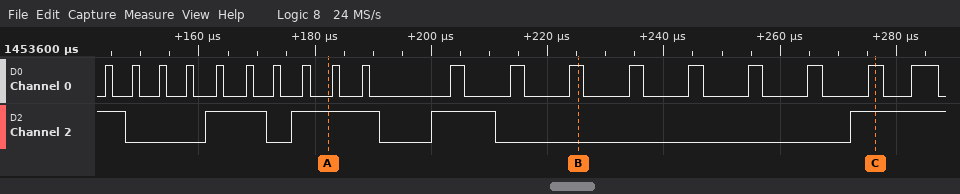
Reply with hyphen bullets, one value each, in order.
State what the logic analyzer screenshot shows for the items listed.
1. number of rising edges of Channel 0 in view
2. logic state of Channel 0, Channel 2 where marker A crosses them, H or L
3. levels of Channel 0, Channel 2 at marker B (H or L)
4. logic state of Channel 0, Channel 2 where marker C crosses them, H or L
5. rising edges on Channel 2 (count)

- 19
- Channel 0=L, Channel 2=H
- Channel 0=H, Channel 2=L
- Channel 0=H, Channel 2=H
- 4
